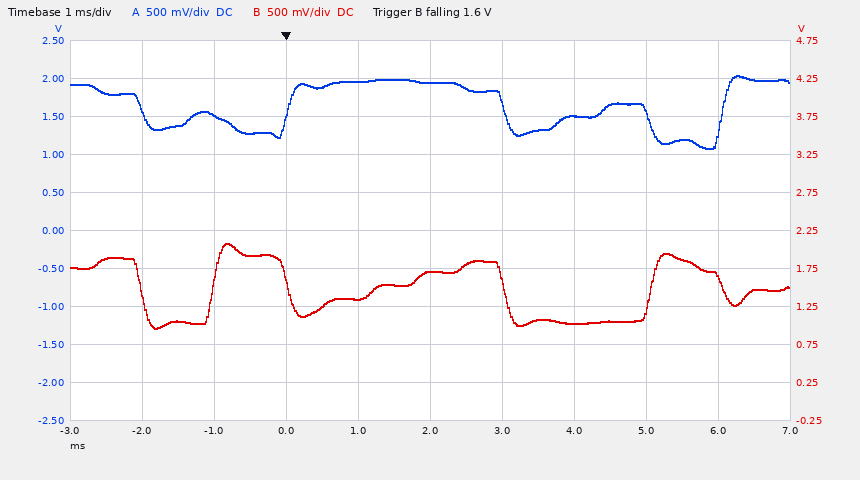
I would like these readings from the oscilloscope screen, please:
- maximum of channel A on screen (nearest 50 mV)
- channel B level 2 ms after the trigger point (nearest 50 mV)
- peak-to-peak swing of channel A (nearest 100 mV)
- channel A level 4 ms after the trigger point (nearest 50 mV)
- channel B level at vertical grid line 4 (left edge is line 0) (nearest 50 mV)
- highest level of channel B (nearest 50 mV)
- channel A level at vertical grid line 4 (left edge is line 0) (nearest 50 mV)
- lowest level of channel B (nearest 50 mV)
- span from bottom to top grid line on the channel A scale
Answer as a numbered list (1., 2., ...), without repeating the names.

1. 2.05 V
2. 1.70 V
3. 1.00 V
4. 1.50 V
5. 1.35 V
6. 2.10 V
7. 1.95 V
8. 950 mV
9. 5 V
